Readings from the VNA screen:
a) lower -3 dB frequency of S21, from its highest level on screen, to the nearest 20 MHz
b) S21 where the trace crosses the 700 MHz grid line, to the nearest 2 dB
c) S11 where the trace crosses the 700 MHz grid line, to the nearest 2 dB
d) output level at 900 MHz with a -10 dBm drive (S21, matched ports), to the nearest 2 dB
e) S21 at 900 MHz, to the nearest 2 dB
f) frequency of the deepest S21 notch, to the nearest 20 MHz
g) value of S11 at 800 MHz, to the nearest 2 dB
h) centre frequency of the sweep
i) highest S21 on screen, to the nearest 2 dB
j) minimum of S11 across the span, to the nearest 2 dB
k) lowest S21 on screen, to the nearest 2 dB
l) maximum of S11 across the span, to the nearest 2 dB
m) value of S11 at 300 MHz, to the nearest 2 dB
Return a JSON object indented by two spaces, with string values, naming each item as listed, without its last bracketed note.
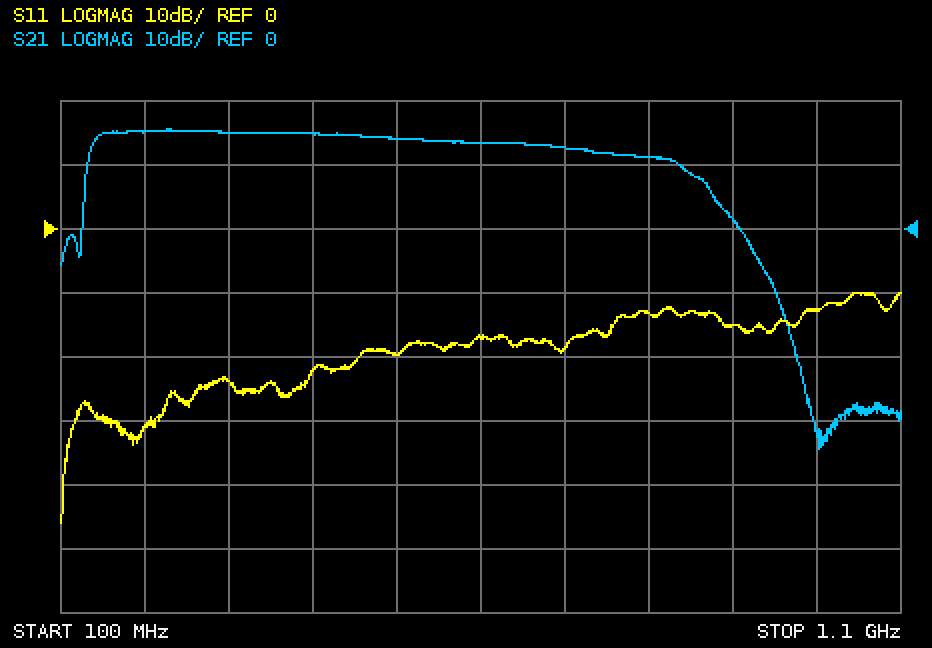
{
  "lower -3 dB frequency of S21, from its highest level on screen, to the nearest 20 MHz": "140 MHz",
  "S21 where the trace crosses the 700 MHz grid line, to the nearest 2 dB": "12 dB",
  "S11 where the trace crosses the 700 MHz grid line, to the nearest 2 dB": "-18 dB",
  "output level at 900 MHz with a -10 dBm drive (S21, matched ports), to the nearest 2 dB": "-8 dBm",
  "S21 at 900 MHz, to the nearest 2 dB": "2 dB",
  "frequency of the deepest S21 notch, to the nearest 20 MHz": "1.00 GHz",
  "value of S11 at 800 MHz, to the nearest 2 dB": "-14 dB",
  "centre frequency of the sweep": "600 MHz",
  "highest S21 on screen, to the nearest 2 dB": "16 dB",
  "minimum of S11 across the span, to the nearest 2 dB": "-46 dB",
  "lowest S21 on screen, to the nearest 2 dB": "-34 dB",
  "maximum of S11 across the span, to the nearest 2 dB": "-10 dB",
  "value of S11 at 300 MHz, to the nearest 2 dB": "-24 dB"
}
